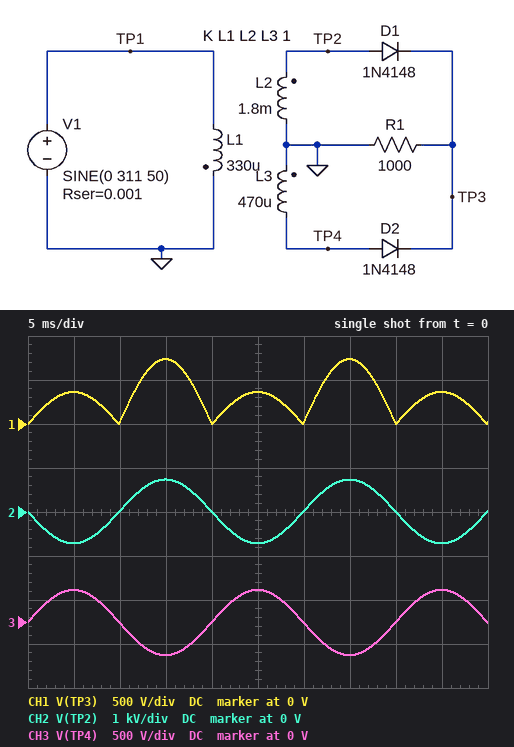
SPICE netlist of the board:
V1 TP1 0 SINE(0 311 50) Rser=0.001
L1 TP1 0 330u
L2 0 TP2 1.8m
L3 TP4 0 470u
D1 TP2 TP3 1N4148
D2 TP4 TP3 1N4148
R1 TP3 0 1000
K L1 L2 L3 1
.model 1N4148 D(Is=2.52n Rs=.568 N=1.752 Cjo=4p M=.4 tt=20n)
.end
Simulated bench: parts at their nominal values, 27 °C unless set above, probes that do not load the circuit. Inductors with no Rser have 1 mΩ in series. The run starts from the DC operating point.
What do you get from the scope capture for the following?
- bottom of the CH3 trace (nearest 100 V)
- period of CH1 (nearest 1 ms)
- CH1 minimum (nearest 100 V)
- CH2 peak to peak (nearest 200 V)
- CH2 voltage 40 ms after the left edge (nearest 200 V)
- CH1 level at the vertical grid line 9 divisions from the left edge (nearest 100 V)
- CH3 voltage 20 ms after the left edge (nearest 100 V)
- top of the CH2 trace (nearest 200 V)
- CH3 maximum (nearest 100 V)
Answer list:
-400 V
20 ms
0 V
1.4 kV
0 V
400 V
0 V
800 V
400 V
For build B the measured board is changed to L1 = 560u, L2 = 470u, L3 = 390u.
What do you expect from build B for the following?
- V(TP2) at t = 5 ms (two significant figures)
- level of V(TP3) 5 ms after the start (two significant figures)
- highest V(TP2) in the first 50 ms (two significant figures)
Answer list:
-280 V
260 V
290 V
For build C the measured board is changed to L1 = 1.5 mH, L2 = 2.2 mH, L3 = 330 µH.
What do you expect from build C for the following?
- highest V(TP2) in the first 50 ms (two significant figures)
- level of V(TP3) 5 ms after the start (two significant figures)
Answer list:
380 V
140 V
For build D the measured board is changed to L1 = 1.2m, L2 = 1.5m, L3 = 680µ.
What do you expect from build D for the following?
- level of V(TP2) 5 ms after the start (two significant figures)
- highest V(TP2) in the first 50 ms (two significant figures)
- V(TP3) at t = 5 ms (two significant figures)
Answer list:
-350 V
350 V
230 V
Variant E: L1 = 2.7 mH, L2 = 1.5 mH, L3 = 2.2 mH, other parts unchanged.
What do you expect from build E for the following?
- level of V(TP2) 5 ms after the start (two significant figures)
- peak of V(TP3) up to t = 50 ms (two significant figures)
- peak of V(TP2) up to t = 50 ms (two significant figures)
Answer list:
-230 V
280 V
230 V
